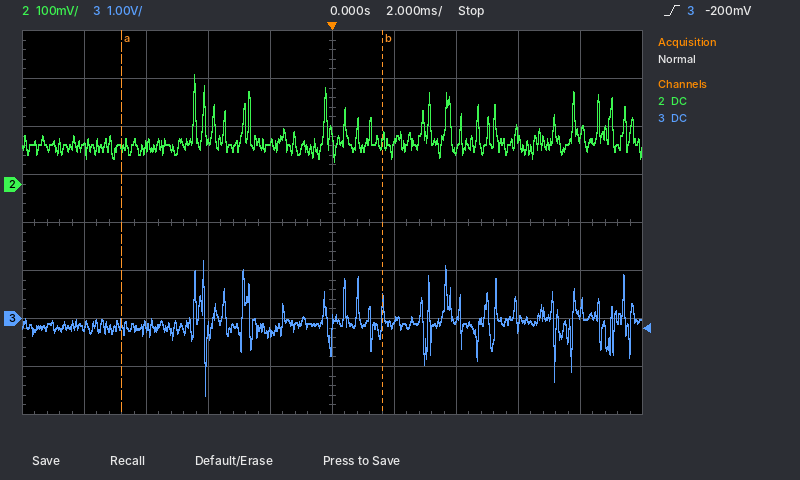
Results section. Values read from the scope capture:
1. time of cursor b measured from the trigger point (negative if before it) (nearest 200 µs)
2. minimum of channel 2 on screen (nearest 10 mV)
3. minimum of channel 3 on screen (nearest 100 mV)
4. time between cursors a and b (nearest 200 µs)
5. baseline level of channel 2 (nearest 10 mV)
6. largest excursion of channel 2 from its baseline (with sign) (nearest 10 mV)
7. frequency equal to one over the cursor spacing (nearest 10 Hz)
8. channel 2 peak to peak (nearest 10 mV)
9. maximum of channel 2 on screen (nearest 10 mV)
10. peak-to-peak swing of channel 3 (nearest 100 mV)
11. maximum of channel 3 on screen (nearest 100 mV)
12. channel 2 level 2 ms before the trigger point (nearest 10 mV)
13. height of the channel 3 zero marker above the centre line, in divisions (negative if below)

+1.6 ms
50 mV
-1.6 V
8.4 ms
80 mV
+150 mV
120 Hz
180 mV
230 mV
2.8 V
1.2 V
90 mV
-2.0 div
